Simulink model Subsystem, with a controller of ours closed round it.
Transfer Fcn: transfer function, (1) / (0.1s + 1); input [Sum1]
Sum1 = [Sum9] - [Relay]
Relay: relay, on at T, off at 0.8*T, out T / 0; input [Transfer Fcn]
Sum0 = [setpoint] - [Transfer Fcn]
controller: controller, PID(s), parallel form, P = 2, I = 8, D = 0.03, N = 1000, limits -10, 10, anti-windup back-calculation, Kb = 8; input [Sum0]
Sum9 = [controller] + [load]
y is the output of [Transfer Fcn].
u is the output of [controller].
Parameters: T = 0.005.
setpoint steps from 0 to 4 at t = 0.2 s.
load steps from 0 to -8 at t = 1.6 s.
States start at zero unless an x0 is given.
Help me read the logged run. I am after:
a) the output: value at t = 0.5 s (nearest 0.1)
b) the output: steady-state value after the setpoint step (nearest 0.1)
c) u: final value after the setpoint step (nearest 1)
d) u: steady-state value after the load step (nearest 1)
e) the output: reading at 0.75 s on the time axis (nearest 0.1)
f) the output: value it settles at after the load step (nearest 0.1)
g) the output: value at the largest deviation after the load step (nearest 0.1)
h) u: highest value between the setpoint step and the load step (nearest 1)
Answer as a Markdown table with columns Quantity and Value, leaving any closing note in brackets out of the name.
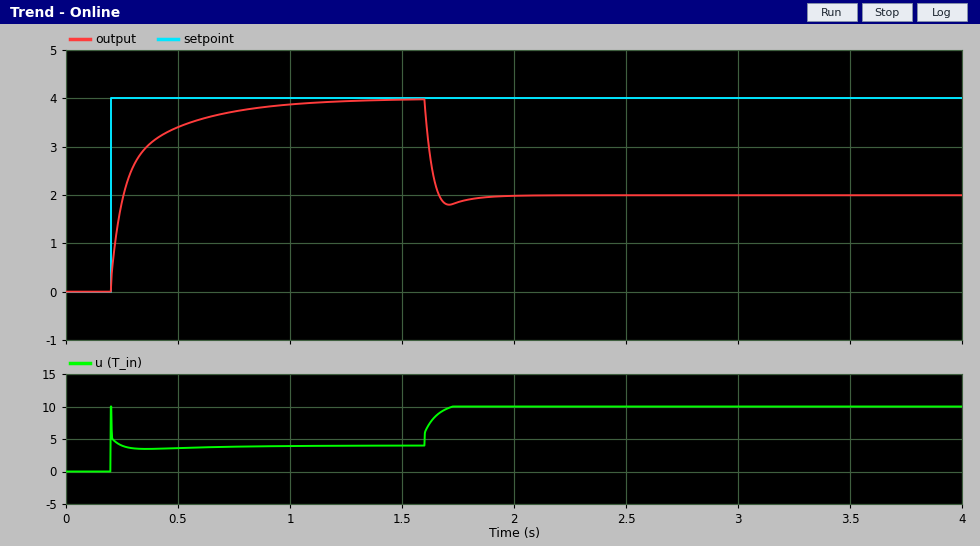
| Quantity | Value |
|---|---|
| the output: value at t = 0.5 s | 3.4 |
| the output: steady-state value after the setpoint step | 4.0 |
| u: final value after the setpoint step | 4 |
| u: steady-state value after the load step | 10 |
| the output: reading at 0.75 s on the time axis | 3.7 |
| the output: value it settles at after the load step | 2.0 |
| the output: value at the largest deviation after the load step | 1.8 |
| u: highest value between the setpoint step and the load step | 10 |
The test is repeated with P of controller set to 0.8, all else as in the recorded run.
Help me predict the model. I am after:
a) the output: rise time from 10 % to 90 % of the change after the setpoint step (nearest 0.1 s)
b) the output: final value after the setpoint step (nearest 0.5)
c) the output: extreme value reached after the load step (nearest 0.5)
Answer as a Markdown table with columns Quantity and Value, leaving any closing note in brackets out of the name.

| Quantity | Value |
|---|---|
| the output: rise time from 10 % to 90 % of the change after the setpoint step | 0.3 s |
| the output: final value after the setpoint step | 4.0 |
| the output: extreme value reached after the load step | 1.0 |
